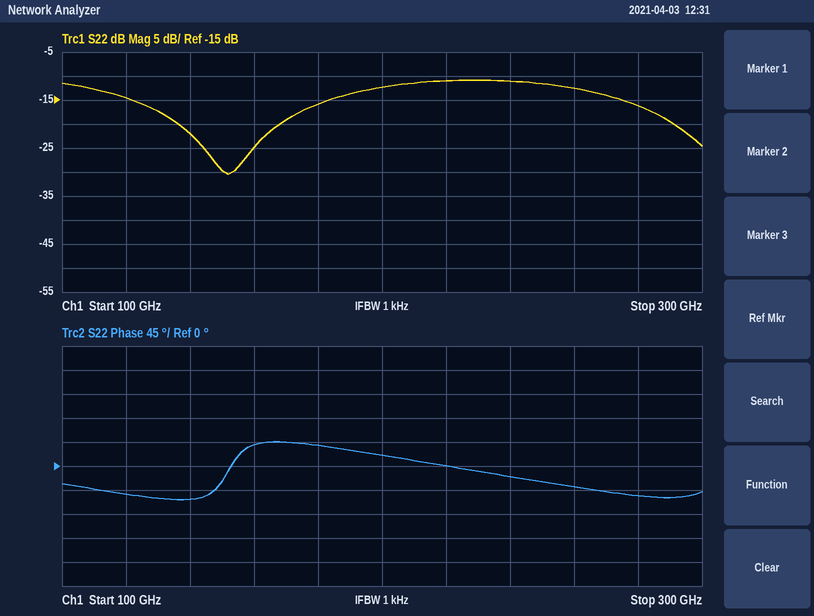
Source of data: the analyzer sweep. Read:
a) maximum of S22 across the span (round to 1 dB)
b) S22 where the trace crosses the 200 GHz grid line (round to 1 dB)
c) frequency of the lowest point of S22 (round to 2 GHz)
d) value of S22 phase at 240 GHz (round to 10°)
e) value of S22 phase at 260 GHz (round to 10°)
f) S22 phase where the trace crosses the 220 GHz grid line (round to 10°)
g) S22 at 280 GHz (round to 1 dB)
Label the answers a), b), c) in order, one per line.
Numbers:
a) -11 dB
b) -12 dB
c) 152 GHz
d) -20°
e) -40°
f) 0°
g) -16 dB
